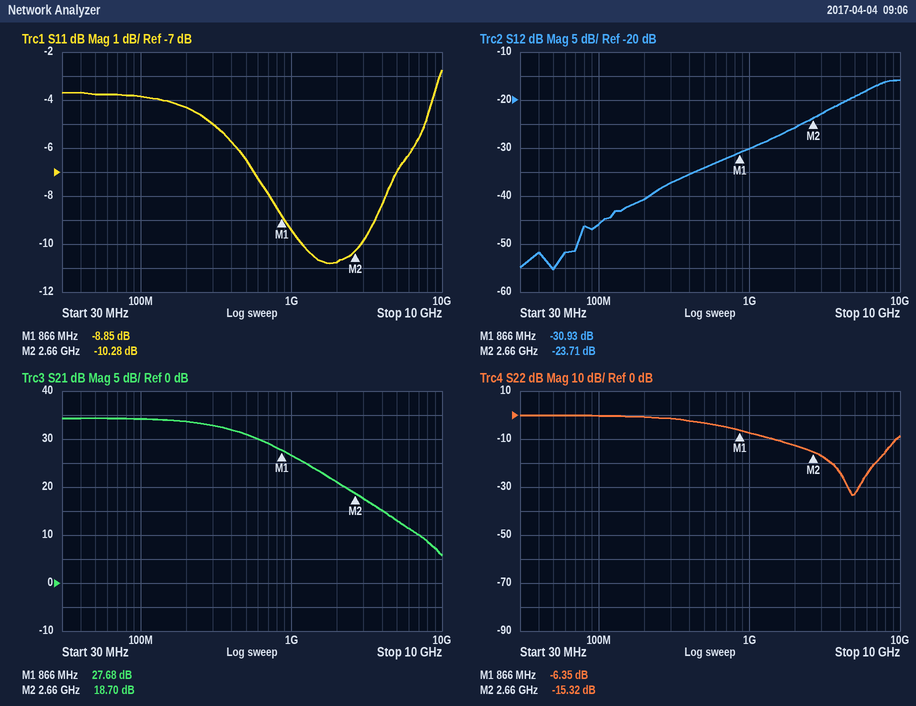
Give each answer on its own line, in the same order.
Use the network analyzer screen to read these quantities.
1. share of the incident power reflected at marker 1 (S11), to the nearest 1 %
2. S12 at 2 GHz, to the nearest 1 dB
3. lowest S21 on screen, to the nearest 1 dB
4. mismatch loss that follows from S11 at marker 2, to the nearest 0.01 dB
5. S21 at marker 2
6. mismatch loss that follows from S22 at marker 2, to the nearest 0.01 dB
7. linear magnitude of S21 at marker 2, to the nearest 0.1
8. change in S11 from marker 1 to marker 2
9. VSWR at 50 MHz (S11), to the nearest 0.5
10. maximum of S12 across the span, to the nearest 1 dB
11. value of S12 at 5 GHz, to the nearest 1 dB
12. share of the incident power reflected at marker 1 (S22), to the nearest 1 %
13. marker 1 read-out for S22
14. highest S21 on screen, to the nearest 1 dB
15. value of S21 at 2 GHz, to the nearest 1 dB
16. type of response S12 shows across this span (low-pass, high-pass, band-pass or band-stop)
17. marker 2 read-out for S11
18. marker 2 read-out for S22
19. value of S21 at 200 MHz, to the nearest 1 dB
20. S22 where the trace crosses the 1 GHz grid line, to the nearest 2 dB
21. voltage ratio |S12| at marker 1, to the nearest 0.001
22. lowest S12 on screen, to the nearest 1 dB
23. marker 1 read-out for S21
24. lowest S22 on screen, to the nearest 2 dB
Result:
13 %
-26 dB
6 dB
0.43 dB
18.70 dB
0.13 dB
8.6
-1.43 dB
4.5
-16 dB
-19 dB
23 %
-6.35 dB
34 dB
21 dB
high-pass
-10.28 dB
-15.32 dB
34 dB
-8 dB
0.028
-55 dB
27.68 dB
-34 dB
